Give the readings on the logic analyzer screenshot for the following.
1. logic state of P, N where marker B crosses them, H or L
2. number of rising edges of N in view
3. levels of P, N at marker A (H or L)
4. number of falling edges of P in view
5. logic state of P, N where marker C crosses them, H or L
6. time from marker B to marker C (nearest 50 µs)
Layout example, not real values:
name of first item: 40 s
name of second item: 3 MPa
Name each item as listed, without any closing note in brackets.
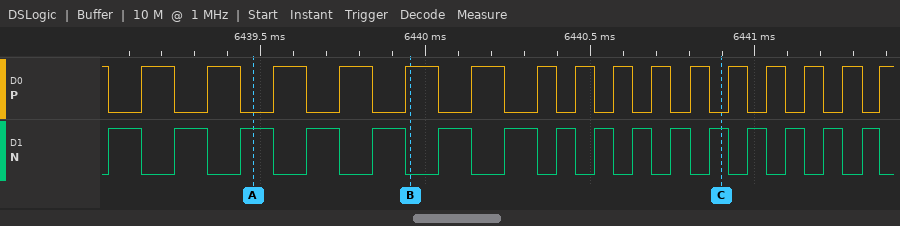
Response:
logic state of P, N where marker B crosses them, H or L: P=H, N=L
number of rising edges of N in view: 16
levels of P, N at marker A: P=L, N=H
number of falling edges of P in view: 16
logic state of P, N where marker C crosses them, H or L: P=L, N=H
time from marker B to marker C: 950 µs
